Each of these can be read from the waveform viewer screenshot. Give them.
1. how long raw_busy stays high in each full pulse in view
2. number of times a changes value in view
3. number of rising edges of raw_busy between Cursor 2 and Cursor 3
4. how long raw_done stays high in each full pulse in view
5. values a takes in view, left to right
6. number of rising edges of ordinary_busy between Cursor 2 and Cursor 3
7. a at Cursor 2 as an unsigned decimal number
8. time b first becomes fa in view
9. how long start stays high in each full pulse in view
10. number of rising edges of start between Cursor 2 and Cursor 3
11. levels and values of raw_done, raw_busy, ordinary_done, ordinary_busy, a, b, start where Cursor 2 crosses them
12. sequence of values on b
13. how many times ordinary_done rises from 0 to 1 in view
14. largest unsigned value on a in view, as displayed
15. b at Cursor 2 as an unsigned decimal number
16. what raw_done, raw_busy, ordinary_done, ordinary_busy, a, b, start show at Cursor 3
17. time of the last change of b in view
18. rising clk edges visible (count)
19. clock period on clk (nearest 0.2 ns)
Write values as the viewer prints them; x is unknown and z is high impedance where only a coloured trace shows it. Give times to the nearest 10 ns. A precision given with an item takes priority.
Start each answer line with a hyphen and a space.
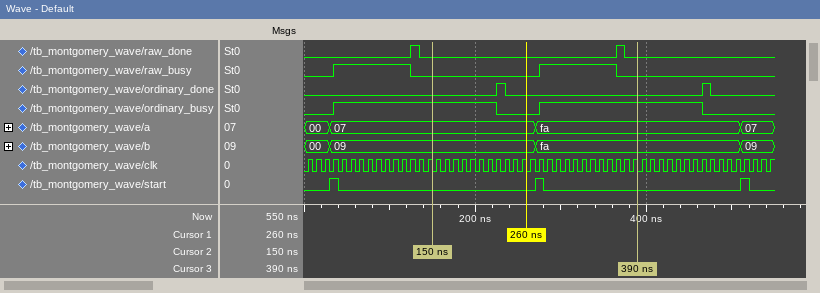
- 90 ns, 90 ns
- 3
- 1
- 10 ns, 10 ns
- 00, 07, fa, 07
- 1
- 7
- 270 ns
- 10 ns, 10 ns, 10 ns
- 1
- raw_done=0, raw_busy=0, ordinary_done=0, ordinary_busy=1, a=07, b=09, start=0
- 00, 09, fa, 09
- 2
- fa
- 9
- raw_done=0, raw_busy=0, ordinary_done=0, ordinary_busy=1, a=fa, b=fa, start=0
- 510 ns
- 55
- 10 ns
